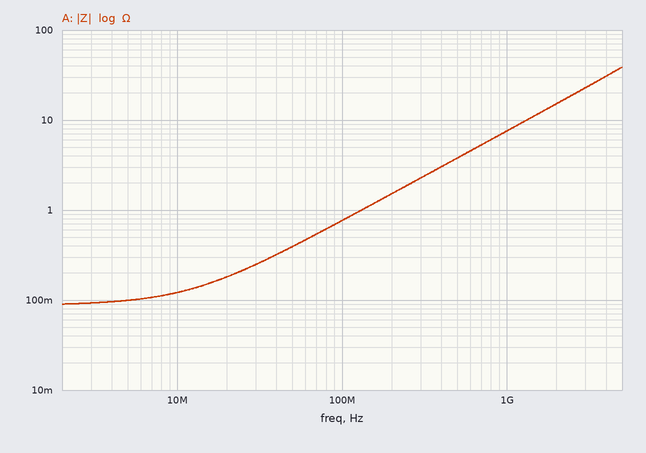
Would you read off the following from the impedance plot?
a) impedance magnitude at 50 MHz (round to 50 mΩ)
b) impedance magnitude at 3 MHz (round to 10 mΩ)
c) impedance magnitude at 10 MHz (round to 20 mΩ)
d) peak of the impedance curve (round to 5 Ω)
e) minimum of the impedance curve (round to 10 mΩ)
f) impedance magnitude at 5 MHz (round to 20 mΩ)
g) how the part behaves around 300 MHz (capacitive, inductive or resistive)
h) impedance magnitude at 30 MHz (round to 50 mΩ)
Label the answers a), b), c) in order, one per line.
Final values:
a) 400 mΩ
b) 90 mΩ
c) 120 mΩ
d) 40 Ω
e) 90 mΩ
f) 100 mΩ
g) inductive
h) 250 mΩ
